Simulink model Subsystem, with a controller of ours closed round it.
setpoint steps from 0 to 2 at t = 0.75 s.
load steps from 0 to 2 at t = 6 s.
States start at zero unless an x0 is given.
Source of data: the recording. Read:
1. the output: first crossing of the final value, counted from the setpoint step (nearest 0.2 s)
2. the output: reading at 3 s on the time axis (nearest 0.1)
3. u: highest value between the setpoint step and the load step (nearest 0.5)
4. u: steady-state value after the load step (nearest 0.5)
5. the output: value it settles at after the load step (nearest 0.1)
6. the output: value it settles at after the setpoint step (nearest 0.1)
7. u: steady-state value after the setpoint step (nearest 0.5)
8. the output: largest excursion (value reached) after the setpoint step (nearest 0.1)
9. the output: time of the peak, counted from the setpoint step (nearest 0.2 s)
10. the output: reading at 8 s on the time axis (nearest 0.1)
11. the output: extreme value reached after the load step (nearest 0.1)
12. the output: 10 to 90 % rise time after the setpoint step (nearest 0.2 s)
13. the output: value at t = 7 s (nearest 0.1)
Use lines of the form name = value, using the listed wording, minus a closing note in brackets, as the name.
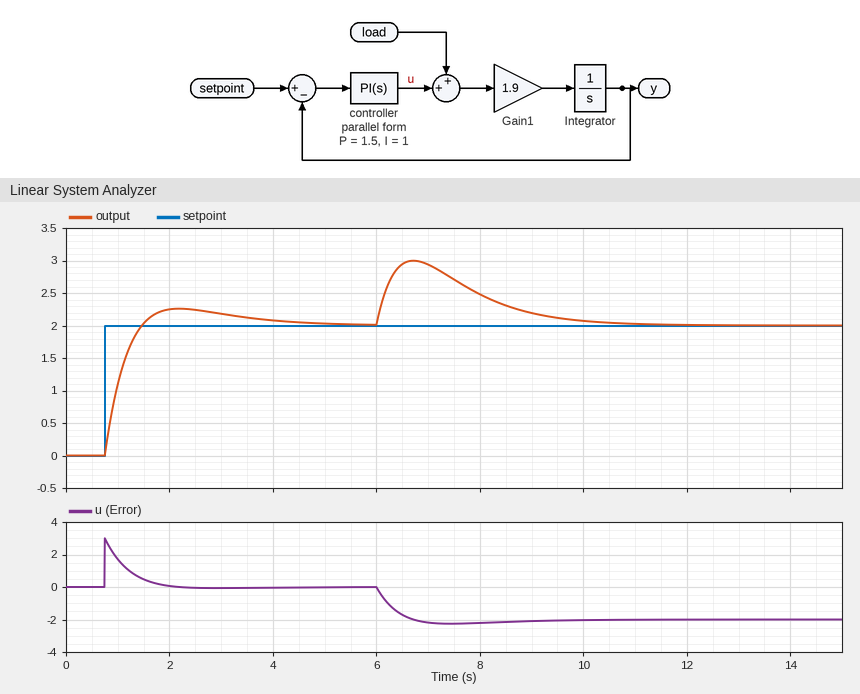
the output: first crossing of the final value, counted from the setpoint step = 0.8 s
the output: reading at 3 s on the time axis = 2.2
u: highest value between the setpoint step and the load step = 3.0
u: steady-state value after the load step = -2.0
the output: value it settles at after the load step = 2.0
the output: value it settles at after the setpoint step = 2.0
u: steady-state value after the setpoint step = 0.0
the output: largest excursion (value reached) after the setpoint step = 2.3
the output: time of the peak, counted from the setpoint step = 1.4 s
the output: reading at 8 s on the time axis = 2.5
the output: extreme value reached after the load step = 3.0
the output: 10 to 90 % rise time after the setpoint step = 0.6 s
the output: value at t = 7 s = 2.9
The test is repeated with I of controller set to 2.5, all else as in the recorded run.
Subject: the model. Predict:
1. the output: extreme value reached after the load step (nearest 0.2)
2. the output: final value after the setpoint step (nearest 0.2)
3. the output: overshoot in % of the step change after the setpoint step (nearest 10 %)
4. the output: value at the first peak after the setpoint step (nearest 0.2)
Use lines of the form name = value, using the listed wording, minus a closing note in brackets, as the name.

the output: extreme value reached after the load step = 2.8
the output: final value after the setpoint step = 2.0
the output: overshoot in % of the step change after the setpoint step = 20 %
the output: value at the first peak after the setpoint step = 2.4
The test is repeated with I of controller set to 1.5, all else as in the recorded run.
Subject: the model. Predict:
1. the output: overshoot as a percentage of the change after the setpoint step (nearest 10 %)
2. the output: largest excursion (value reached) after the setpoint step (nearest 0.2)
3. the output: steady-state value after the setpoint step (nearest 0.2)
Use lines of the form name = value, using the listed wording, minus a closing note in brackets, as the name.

the output: overshoot as a percentage of the change after the setpoint step = 20 %
the output: largest excursion (value reached) after the setpoint step = 2.4
the output: steady-state value after the setpoint step = 2.0
